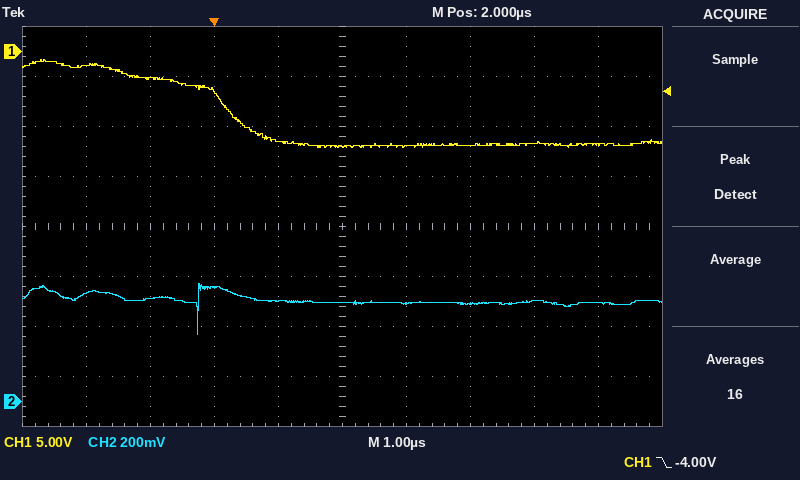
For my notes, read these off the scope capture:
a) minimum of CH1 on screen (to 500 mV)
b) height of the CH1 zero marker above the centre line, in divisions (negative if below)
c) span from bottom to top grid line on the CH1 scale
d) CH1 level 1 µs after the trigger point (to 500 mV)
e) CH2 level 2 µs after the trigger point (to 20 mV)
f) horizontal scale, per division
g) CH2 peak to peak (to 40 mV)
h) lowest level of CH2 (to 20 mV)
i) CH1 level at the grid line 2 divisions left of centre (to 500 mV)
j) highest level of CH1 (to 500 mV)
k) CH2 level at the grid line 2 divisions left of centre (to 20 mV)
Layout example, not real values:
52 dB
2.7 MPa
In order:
-9.5 V
+3.5 div
40 V
-9.0 V
400 mV
1 µs
200 mV
260 mV
-4.0 V
-1.0 V
460 mV
